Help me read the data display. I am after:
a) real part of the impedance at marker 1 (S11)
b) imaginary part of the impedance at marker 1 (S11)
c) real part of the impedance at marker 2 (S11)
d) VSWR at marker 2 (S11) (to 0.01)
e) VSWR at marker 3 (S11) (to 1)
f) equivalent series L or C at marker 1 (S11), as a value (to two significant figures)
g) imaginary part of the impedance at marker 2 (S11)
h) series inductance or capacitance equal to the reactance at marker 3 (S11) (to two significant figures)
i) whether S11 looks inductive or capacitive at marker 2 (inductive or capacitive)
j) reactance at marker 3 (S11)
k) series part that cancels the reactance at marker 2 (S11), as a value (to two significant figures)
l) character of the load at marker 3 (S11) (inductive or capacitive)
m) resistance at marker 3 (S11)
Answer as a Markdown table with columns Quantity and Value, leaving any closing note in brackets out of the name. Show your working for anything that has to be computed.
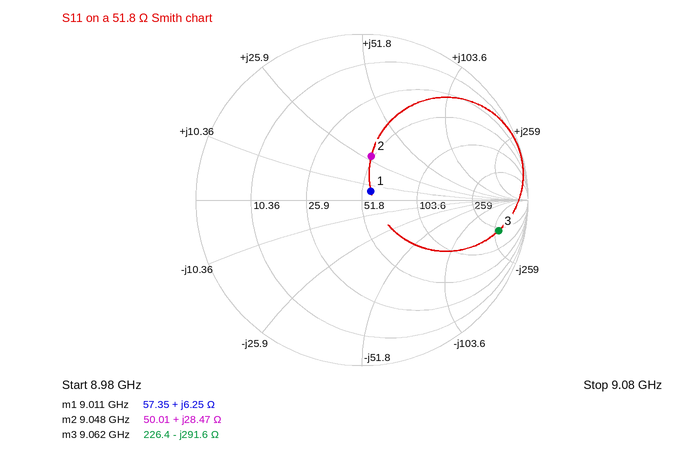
| Quantity | Value |
|---|---|
| real part of the impedance at marker 1 | 57.35 Ω |
| imaginary part of the impedance at marker 1 | +6.25 Ω |
| real part of the impedance at marker 2 | 50.01 Ω |
| VSWR at marker 2 (S11) | 1.74 |
| VSWR at marker 3 (S11) | 12 |
| equivalent series L or C at marker 1 (S11), as a value | L = 6.25 Ω/(2π × 9.011 GHz) ≈ 110 pH |
| imaginary part of the impedance at marker 2 | +28.47 Ω |
| series inductance or capacitance equal to the reactance at marker 3 (S11) | C = 1/(2π × 9.062 GHz × 291.6 Ω) ≈ 60 fF |
| whether S11 looks inductive or capacitive at marker 2 | inductive |
| reactance at marker 3 | -291.6 Ω |
| series part that cancels the reactance at marker 2 (S11), as a value | C = 1/(2π × 9.048 GHz × 28.47 Ω) ≈ 618 fF, so 620 fF to two significant figures |
| character of the load at marker 3 (S11) | capacitive |
| resistance at marker 3 | 226.4 Ω |
